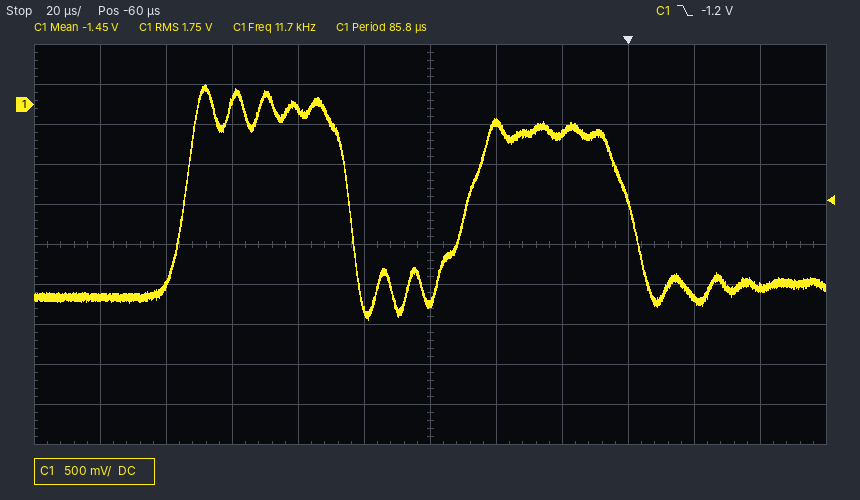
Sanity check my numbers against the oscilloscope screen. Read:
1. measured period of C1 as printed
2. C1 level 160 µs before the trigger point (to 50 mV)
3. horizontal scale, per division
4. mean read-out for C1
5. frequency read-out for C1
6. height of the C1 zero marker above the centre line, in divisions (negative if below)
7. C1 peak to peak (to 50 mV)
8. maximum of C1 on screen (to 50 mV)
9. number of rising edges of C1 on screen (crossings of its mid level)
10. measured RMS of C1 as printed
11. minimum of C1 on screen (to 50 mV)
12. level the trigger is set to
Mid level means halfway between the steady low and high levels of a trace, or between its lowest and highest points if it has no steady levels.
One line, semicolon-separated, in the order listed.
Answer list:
85.8 µs; -2.40 V; 20 µs; -1.45 V; 11.7 kHz; +3.5 div; 2.95 V; 250 mV; 2; 1.75 V; -2.70 V; -1.2 V
